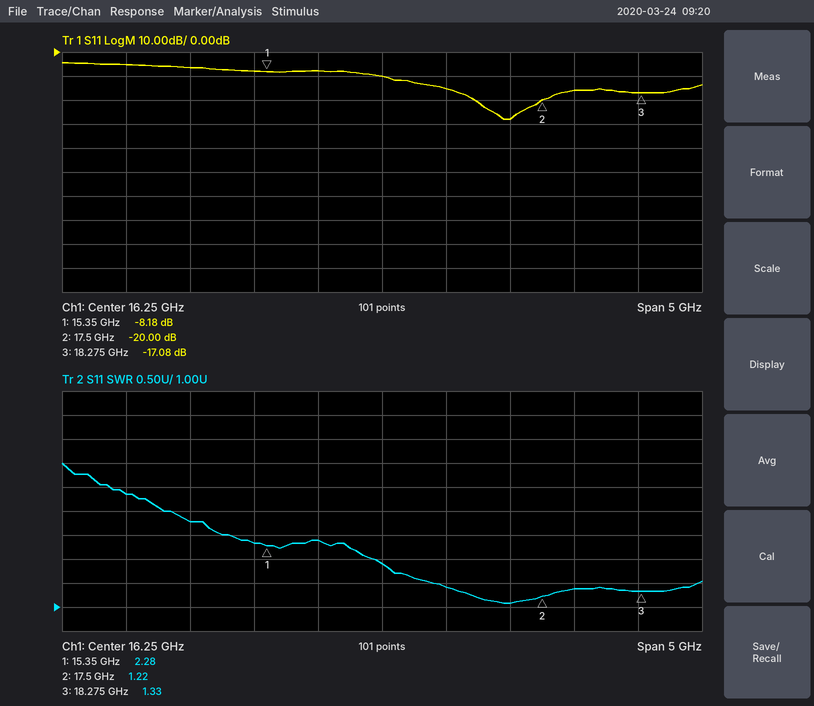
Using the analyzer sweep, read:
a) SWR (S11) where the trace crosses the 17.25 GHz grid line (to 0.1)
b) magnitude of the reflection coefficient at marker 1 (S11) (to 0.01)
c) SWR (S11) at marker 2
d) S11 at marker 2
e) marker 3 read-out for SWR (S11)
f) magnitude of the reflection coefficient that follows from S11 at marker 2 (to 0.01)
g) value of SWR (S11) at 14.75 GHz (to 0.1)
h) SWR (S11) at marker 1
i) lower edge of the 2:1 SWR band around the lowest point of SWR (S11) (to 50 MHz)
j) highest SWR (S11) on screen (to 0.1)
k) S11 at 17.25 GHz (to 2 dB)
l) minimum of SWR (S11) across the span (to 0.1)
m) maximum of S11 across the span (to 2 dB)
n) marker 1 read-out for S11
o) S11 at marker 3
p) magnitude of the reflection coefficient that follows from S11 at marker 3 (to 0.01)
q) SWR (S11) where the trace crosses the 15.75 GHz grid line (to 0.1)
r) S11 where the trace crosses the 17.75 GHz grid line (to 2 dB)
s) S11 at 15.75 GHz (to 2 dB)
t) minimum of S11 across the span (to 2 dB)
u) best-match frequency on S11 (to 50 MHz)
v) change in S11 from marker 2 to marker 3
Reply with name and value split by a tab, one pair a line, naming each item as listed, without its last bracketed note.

SWR (S11) where the trace crosses the 17.25 GHz grid line	1.1
magnitude of the reflection coefficient at marker 1 (S11)	0.39
SWR (S11) at marker 2	1.22
S11 at marker 2	-20.00 dB
marker 3 read-out for SWR	1.33
magnitude of the reflection coefficient that follows from S11 at marker 2	0.10
value of SWR (S11) at 14.75 GHz	2.8
SWR (S11) at marker 1	2.28
lower edge of the 2:1 SWR band around the lowest point of SWR (S11)	16.20 GHz
highest SWR (S11) on screen	4.0
S11 at 17.25 GHz	-28 dB
minimum of SWR (S11) across the span	1.1
maximum of S11 across the span	-4 dB
marker 1 read-out for S11	-8.18 dB
S11 at marker 3	-17.08 dB
magnitude of the reflection coefficient that follows from S11 at marker 3	0.14
SWR (S11) where the trace crosses the 15.75 GHz grid line	2.4
S11 where the trace crosses the 17.75 GHz grid line	-16 dB
S11 at 15.75 GHz	-8 dB
minimum of S11 across the span	-28 dB
best-match frequency on S11	17.20 GHz
change in S11 from marker 2 to marker 3	2.92 dB
